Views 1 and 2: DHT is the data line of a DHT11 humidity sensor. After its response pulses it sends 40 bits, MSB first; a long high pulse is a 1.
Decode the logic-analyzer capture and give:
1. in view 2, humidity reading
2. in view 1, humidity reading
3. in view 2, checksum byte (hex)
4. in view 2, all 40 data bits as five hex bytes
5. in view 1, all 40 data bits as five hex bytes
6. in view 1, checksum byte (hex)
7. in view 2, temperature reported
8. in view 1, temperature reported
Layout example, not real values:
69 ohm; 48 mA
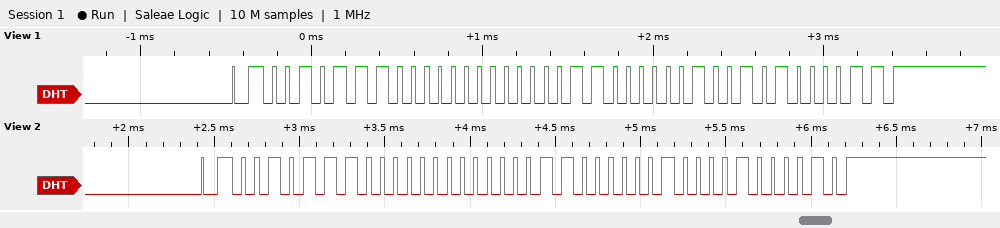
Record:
46 %; 46 %; 0x42; 2E 00 0C 08 42; 2E 00 0C 09 43; 0x43; 12.8 °C; 12.9 °C
